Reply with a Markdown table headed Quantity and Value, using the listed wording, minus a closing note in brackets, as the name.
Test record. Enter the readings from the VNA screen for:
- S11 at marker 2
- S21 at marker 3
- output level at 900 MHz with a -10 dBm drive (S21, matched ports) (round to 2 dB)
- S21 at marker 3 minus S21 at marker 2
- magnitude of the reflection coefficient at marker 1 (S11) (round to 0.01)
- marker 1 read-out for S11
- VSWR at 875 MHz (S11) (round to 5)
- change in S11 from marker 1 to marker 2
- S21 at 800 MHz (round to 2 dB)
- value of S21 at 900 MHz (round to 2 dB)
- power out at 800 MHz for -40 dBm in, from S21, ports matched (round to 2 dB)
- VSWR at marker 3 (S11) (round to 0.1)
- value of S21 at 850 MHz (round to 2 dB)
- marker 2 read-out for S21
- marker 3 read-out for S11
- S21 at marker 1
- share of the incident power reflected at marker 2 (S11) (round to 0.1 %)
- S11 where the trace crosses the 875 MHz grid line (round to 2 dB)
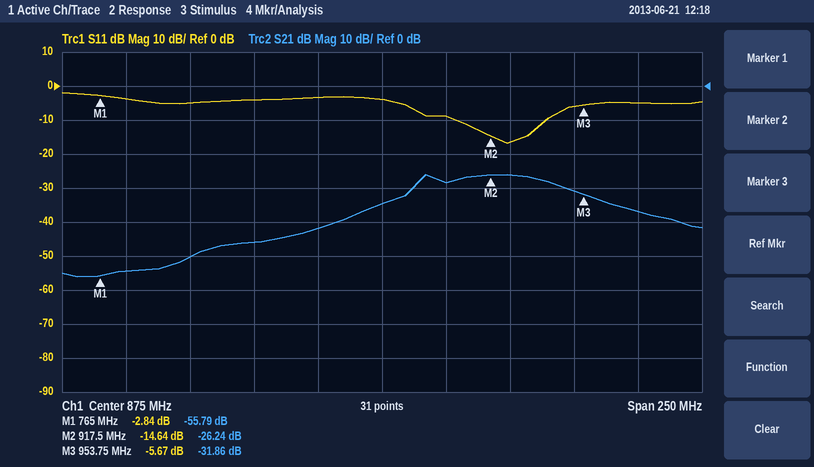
| Quantity | Value |
|---|---|
| S11 at marker 2 | -14.64 dB |
| S21 at marker 3 | -31.86 dB |
| output level at 900 MHz with a -10 dBm drive (S21, matched ports) | -38 dBm |
| S21 at marker 3 minus S21 at marker 2 | -5.62 dB |
| magnitude of the reflection coefficient at marker 1 (S11) | 0.72 |
| marker 1 read-out for S11 | -2.84 dB |
| VSWR at 875 MHz (S11) | 5 |
| change in S11 from marker 1 to marker 2 | -11.80 dB |
| S21 at 800 MHz | -50 dB |
| value of S21 at 900 MHz | -28 dB |
| power out at 800 MHz for -40 dBm in, from S21, ports matched | -90 dBm |
| VSWR at marker 3 (S11) | 3.2 |
| value of S21 at 850 MHz | -42 dB |
| marker 2 read-out for S21 | -26.24 dB |
| marker 3 read-out for S11 | -5.67 dB |
| S21 at marker 1 | -55.79 dB |
| share of the incident power reflected at marker 2 (S11) | 3.4 % |
| S11 where the trace crosses the 875 MHz grid line | -4 dB |
